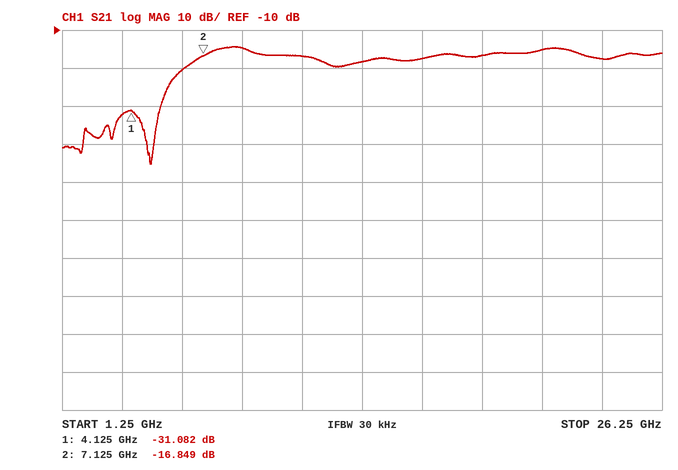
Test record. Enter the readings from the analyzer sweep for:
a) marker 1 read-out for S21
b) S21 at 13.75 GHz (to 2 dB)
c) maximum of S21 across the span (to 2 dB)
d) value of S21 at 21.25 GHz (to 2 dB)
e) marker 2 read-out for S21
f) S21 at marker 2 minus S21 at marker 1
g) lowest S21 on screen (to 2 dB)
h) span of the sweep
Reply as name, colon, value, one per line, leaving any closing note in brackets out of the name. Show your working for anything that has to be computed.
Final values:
marker 1 read-out for S21: -31.082 dB
S21 at 13.75 GHz: -18 dB
maximum of S21 across the span: -14 dB
value of S21 at 21.25 GHz: -16 dB
marker 2 read-out for S21: -16.849 dB
S21 at marker 2 minus S21 at marker 1: -16.849 − (-31.082) = 14.233 dB
lowest S21 on screen: -46 dB
span of the sweep: 25 GHz
